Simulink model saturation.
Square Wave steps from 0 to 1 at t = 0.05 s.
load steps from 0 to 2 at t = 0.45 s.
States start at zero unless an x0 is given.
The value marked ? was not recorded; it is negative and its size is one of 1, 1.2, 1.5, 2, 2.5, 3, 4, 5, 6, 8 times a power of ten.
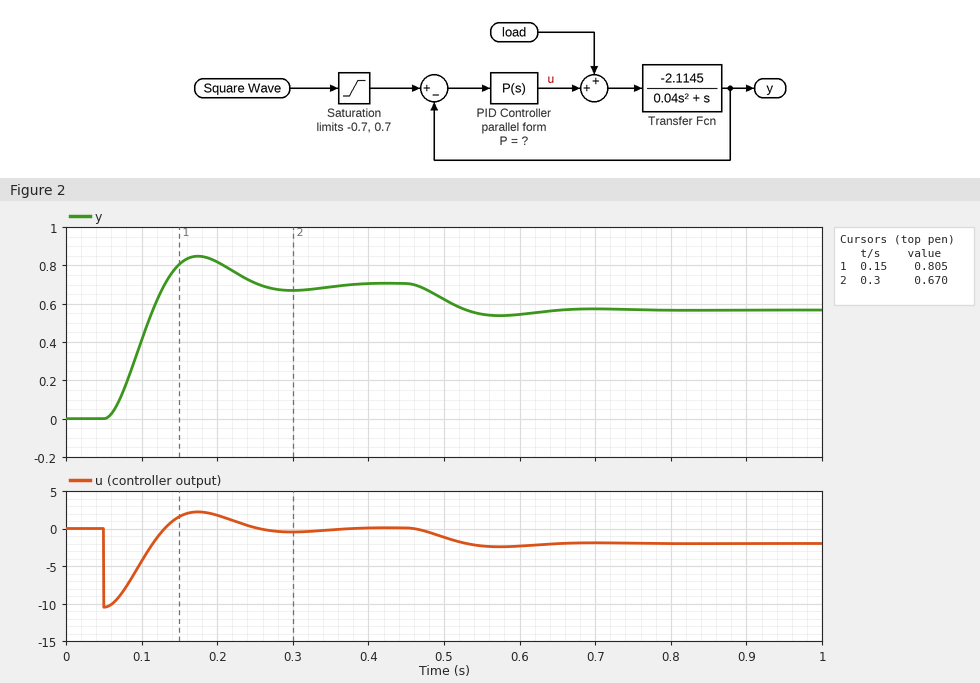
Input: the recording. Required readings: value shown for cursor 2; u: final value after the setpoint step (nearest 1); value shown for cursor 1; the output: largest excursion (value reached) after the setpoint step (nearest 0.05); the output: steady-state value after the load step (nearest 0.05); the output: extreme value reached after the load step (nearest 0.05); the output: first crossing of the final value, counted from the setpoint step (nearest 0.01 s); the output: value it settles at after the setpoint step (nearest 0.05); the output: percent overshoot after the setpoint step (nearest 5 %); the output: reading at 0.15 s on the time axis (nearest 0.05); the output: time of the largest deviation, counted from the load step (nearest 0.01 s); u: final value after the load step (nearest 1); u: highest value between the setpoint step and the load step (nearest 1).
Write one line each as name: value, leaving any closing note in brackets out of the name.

value shown for cursor 2: 0.670
u: final value after the setpoint step: 0
value shown for cursor 1: 0.805
the output: largest excursion (value reached) after the setpoint step: 0.85
the output: steady-state value after the load step: 0.55
the output: extreme value reached after the load step: 0.55
the output: first crossing of the final value, counted from the setpoint step: 0.08 s
the output: value it settles at after the setpoint step: 0.70
the output: percent overshoot after the setpoint step: 20 %
the output: reading at 0.15 s on the time axis: 0.80
the output: time of the largest deviation, counted from the load step: 0.12 s
u: final value after the load step: -2
u: highest value between the setpoint step and the load step: 2
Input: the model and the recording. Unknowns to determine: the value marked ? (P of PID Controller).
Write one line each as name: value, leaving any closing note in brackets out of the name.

the value marked ?: -15
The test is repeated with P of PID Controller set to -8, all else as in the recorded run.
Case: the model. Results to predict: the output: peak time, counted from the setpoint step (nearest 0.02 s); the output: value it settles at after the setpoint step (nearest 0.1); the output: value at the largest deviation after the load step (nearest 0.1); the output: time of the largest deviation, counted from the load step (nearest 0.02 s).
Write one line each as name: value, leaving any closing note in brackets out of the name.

the output: peak time, counted from the setpoint step: 0.20 s
the output: value it settles at after the setpoint step: 0.7
the output: value at the largest deviation after the load step: 0.4
the output: time of the largest deviation, counted from the load step: 0.20 s
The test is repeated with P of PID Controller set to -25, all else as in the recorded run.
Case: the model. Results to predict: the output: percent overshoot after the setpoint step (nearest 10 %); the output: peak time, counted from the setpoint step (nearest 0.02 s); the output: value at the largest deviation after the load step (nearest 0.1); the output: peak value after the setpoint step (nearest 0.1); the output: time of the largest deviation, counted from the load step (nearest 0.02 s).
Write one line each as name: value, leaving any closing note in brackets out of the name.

the output: percent overshoot after the setpoint step: 30 %
the output: peak time, counted from the setpoint step: 0.10 s
the output: value at the largest deviation after the load step: 0.6
the output: peak value after the setpoint step: 0.9
the output: time of the largest deviation, counted from the load step: 0.10 s
